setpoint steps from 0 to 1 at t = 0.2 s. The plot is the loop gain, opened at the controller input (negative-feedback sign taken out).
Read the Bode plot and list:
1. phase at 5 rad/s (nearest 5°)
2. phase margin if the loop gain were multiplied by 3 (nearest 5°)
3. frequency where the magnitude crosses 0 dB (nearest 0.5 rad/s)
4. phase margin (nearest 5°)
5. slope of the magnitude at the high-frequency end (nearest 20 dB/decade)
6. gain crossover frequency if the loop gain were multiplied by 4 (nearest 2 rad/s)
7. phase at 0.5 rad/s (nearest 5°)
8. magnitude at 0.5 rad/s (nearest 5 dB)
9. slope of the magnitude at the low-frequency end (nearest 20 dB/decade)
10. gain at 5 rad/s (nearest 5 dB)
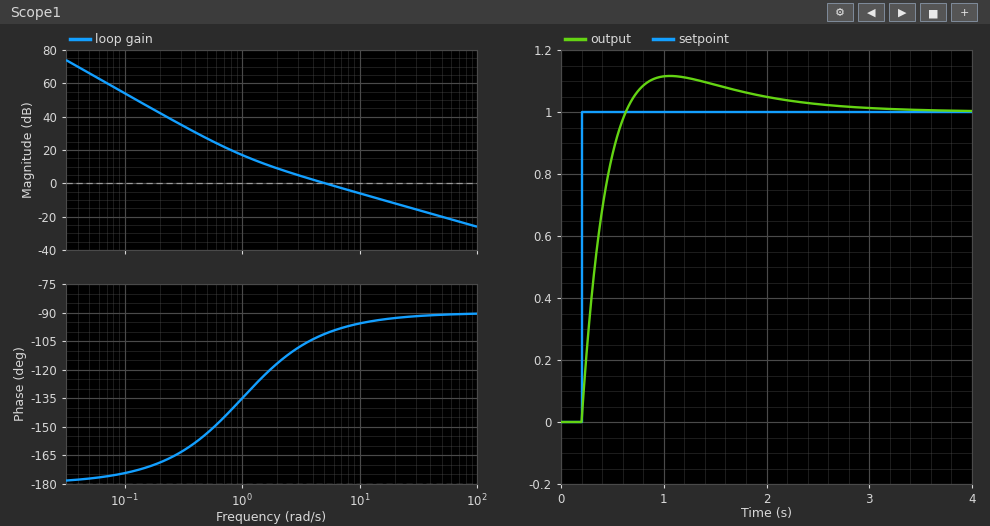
-100°
85°
5.0 rad/s
80°
-20 dB/decade
20 rad/s
-155°
25 dB
-40 dB/decade
0 dB
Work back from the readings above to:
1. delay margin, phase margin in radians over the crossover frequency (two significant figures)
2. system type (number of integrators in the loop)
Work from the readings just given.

0.28 s
2
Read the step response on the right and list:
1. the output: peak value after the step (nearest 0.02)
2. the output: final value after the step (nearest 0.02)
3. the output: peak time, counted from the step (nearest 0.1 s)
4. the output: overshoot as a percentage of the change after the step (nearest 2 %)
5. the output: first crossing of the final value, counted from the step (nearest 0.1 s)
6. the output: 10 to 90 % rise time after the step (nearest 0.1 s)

1.12
1.00
0.9 s
12 %
0.4 s
0.3 s
